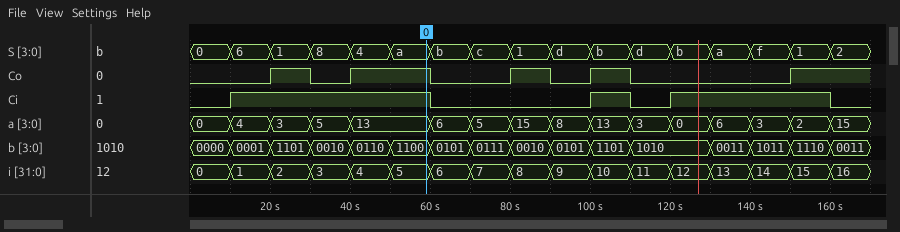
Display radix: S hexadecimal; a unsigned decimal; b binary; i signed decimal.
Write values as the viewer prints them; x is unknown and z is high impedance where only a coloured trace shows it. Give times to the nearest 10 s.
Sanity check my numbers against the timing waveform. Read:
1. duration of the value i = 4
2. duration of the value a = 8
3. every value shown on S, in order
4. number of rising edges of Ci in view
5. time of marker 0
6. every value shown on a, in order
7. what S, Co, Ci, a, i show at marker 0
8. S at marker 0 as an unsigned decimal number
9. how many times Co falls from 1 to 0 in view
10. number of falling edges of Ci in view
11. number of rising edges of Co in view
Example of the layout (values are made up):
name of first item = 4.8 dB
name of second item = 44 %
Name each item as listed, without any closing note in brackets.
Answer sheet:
duration of the value i = 4 = 10 s
duration of the value a = 8 = 10 s
every value shown on S, in order = 0, 6, 1, 8, 4, a, b, c, 1, d, b, d, b, a, f, 1, 2
number of rising edges of Ci in view = 3
time of marker 0 = 60 s
every value shown on a, in order = 0, 4, 3, 5, 13, 6, 5, 15, 8, 13, 3, 0, 6, 3, 2, 15
what S, Co, Ci, a, i show at marker 0 = S=a, Co=1, Ci=1, a=13, i=5
S at marker 0 as an unsigned decimal number = 10
how many times Co falls from 1 to 0 in view = 4
number of falling edges of Ci in view = 3
number of rising edges of Co in view = 5
